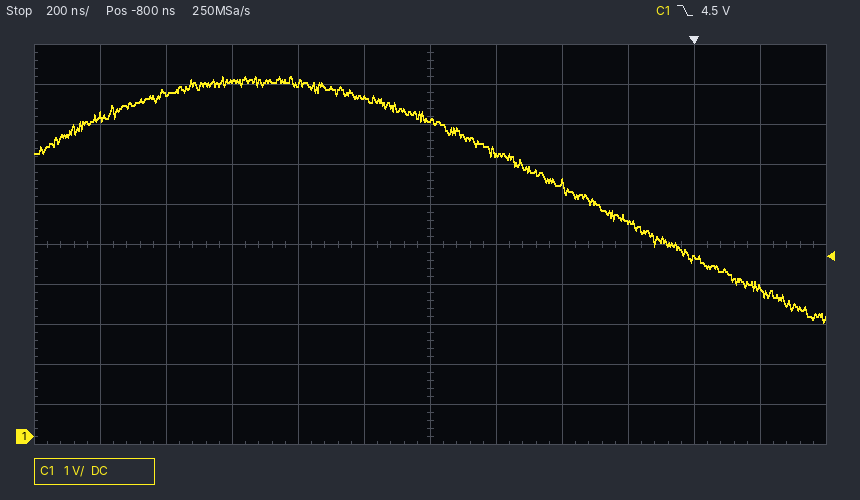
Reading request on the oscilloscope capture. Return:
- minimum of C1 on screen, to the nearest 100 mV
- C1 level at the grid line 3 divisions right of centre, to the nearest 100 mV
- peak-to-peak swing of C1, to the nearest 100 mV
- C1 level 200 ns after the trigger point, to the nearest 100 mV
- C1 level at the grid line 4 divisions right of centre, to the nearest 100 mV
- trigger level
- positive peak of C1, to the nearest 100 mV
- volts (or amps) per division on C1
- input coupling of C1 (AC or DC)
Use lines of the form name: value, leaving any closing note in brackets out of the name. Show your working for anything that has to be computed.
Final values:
minimum of C1 on screen, to the nearest 100 mV: 2.8 V
C1 level at the grid line 3 divisions right of centre, to the nearest 100 mV: 5.4 V
peak-to-peak swing of C1, to the nearest 100 mV: 9.0 V − (2.8 V) = 6.2 V
C1 level 200 ns after the trigger point, to the nearest 100 mV: 3.7 V
C1 level at the grid line 4 divisions right of centre, to the nearest 100 mV: 4.4 V
trigger level: 4.5 V
positive peak of C1, to the nearest 100 mV: 9.0 V
volts (or amps) per division on C1: 1 V
input coupling of C1: DC
